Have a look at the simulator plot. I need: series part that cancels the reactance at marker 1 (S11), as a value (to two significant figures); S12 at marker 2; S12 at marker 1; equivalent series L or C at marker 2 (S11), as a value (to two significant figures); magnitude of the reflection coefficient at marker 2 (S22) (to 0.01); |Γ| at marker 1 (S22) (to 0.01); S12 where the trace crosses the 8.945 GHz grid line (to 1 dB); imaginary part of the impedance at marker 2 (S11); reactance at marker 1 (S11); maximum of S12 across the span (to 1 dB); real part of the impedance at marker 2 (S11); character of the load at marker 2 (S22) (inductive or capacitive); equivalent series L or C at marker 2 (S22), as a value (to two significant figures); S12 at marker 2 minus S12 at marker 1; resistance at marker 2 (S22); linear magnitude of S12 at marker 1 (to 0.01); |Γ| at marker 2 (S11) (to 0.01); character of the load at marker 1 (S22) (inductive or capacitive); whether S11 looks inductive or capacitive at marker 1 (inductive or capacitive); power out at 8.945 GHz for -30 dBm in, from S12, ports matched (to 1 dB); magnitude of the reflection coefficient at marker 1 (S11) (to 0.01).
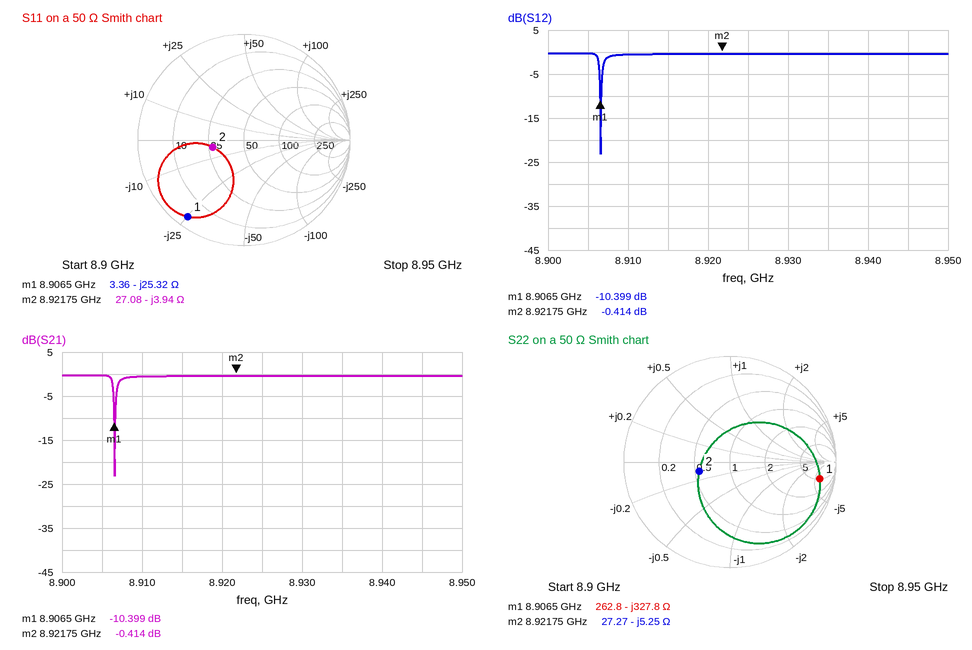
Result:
450 pH
-0.414 dB
-10.399 dB
4.5 pF
0.30
0.86
0 dB
-3.94 Ω
-25.32 Ω
0 dB
27.08 Ω
capacitive
3.4 pF
9.985 dB
27.27 Ω
0.30
0.30
capacitive
capacitive
-30 dBm
0.90
